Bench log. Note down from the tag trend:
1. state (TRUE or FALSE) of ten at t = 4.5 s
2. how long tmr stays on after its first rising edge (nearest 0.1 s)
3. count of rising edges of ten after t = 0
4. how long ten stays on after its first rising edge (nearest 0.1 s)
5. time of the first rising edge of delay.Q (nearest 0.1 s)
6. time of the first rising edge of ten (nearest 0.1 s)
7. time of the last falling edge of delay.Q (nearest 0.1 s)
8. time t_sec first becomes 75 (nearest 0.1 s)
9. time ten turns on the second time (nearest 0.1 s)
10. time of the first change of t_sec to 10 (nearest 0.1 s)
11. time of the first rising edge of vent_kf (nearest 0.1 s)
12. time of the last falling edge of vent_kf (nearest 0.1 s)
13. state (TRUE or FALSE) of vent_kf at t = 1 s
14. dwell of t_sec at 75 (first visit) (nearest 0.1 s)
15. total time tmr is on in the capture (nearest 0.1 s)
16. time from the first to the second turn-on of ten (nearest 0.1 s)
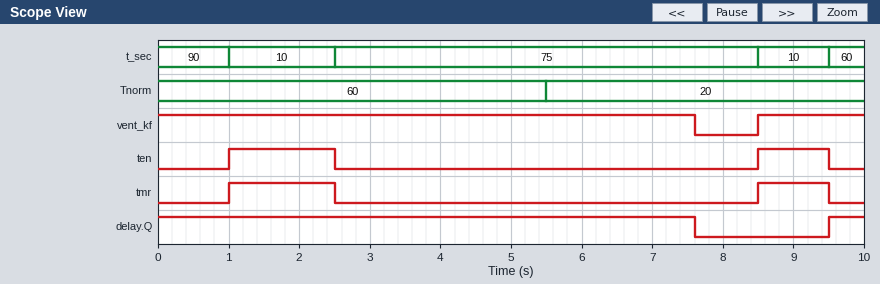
FALSE
1.5 s
2
1.5 s
9.5 s
1.0 s
7.6 s
2.5 s
8.5 s
1.0 s
8.5 s
7.6 s
TRUE
6.0 s
2.5 s
7.5 s
